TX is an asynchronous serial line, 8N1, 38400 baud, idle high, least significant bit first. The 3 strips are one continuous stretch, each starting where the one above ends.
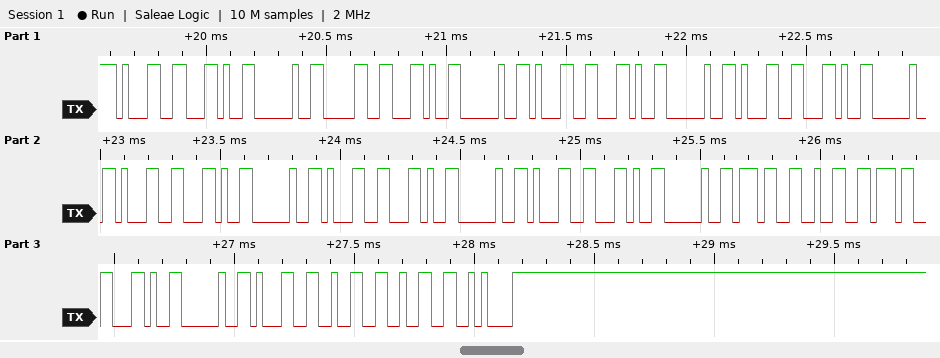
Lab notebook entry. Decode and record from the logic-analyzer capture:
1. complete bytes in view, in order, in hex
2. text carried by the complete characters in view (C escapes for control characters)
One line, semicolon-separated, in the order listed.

0x31 0x2C 0x20 0x30 0x2C 0x20 0x31 0x2C 0x20 0x31 0x2C 0x20 0x31 0x2C 0x20 0x31 0x2C 0x20 0x31 0x2C 0x20 0x37 0x32 0x37 0x2C 0x20 0x31 0x32 0x32 0x0A; "1, 0, 1, 1, 1, 1, 1, 727, 122\n"
